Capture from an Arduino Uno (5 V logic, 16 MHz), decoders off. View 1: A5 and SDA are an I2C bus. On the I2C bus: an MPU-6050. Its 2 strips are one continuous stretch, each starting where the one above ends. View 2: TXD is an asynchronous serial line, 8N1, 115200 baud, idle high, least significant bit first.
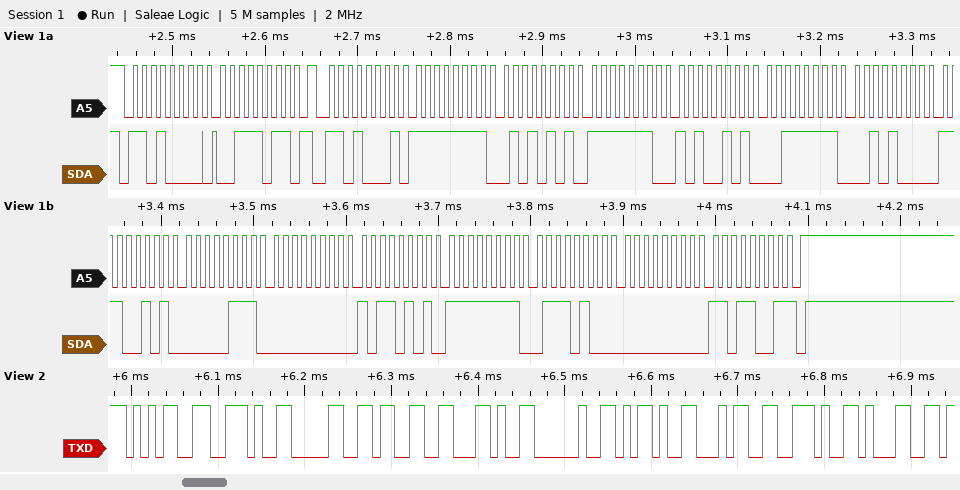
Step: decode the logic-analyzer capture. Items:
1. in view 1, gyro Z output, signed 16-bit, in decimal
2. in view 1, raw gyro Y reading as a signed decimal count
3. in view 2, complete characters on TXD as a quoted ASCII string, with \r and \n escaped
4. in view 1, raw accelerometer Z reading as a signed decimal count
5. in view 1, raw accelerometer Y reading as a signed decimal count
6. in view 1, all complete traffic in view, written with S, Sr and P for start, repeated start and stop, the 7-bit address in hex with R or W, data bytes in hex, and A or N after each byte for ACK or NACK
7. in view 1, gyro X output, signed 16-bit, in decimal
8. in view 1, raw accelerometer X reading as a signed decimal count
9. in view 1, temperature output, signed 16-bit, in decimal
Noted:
217
-140
"5.03, -4.1"
16168
-347
S 68W A 3B A Sr 68R A FF A 55 A FE A A5 A 3F A 28 A E5 A 07 A 00 A B5 A FF A 74 A 00 A D9 N P
181
-171
-6905
